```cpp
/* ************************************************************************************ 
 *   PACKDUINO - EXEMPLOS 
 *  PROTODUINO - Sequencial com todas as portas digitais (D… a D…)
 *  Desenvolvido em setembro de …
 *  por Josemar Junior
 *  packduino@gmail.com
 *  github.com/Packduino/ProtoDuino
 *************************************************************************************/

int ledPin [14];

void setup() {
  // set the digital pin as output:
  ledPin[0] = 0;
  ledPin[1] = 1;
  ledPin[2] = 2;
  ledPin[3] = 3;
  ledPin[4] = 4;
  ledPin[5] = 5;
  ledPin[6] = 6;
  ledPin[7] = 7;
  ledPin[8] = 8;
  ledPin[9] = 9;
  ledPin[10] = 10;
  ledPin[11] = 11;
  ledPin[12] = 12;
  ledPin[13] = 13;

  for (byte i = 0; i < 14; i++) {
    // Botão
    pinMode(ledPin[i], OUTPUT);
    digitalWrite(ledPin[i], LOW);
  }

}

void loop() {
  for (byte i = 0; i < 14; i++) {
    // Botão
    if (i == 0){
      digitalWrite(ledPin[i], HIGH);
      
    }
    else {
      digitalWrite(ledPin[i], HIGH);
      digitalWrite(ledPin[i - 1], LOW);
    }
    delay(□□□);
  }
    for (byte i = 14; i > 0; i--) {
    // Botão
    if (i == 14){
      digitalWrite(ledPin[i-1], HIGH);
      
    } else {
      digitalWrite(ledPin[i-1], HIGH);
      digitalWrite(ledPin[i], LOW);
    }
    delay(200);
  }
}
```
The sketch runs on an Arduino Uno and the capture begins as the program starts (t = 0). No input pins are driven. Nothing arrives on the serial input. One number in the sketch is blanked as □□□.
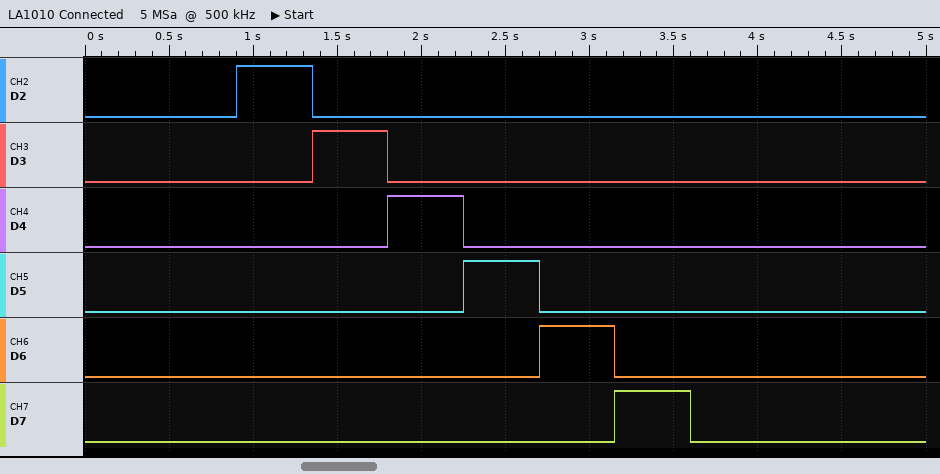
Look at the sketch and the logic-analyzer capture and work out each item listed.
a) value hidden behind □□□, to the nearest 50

450
